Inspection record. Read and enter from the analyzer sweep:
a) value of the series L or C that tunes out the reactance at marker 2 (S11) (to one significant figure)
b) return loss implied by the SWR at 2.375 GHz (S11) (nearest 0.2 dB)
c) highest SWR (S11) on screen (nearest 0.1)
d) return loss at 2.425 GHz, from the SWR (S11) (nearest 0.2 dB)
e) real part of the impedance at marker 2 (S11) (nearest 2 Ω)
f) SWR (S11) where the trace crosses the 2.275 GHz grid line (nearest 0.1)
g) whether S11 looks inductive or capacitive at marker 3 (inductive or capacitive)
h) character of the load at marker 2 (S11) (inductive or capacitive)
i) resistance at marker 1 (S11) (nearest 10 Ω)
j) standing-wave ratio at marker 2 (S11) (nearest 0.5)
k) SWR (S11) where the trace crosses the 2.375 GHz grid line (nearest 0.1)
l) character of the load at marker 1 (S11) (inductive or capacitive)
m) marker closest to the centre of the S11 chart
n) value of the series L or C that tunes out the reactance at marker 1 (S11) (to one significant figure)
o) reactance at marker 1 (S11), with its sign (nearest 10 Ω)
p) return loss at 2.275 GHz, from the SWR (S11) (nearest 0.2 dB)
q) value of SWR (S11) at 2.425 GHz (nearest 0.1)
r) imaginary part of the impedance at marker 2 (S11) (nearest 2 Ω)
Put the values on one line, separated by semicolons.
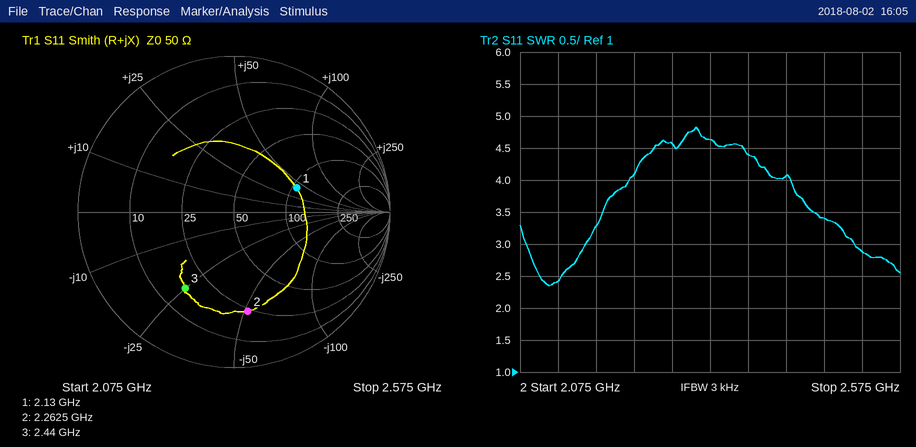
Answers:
4 nH; 4.0 dB; 4.8; 4.4 dB; 24 Ω; 4.6; capacitive; capacitive; 110 Ω; 4.5; 4.4; inductive; marker 1; 2 pF; +40 Ω; 3.8 dB; 4.1; -52 Ω
